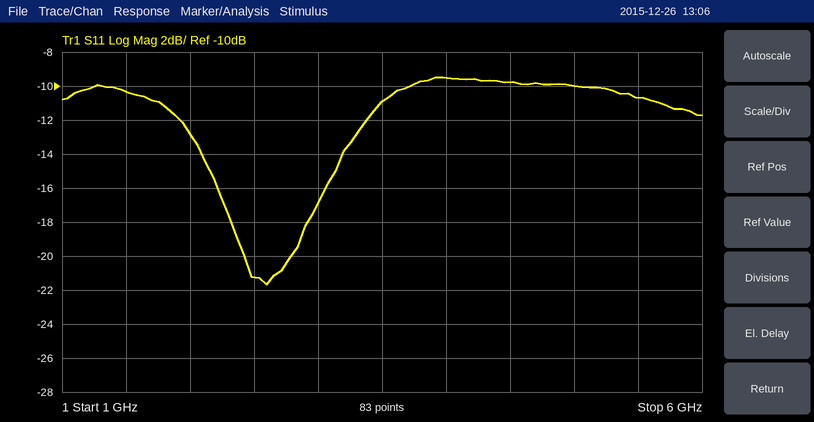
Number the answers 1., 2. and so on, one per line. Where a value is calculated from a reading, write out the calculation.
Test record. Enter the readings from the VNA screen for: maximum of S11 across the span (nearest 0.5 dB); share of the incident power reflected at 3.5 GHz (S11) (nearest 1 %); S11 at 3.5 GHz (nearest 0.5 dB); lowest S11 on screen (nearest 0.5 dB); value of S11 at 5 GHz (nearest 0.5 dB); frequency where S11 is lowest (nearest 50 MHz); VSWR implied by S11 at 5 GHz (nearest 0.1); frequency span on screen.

1. -9.5 dB
2. 10^(-11/10) ≈ 8 %
3. -11.0 dB
4. -21.5 dB
5. -10.0 dB
6. 2.60 GHz
7. |Γ| = 10^(-10/20) = 0.3162; VSWR = (1 + 0.3162)/(1 − 0.3162) ≈ 1.9
8. 5 GHz
